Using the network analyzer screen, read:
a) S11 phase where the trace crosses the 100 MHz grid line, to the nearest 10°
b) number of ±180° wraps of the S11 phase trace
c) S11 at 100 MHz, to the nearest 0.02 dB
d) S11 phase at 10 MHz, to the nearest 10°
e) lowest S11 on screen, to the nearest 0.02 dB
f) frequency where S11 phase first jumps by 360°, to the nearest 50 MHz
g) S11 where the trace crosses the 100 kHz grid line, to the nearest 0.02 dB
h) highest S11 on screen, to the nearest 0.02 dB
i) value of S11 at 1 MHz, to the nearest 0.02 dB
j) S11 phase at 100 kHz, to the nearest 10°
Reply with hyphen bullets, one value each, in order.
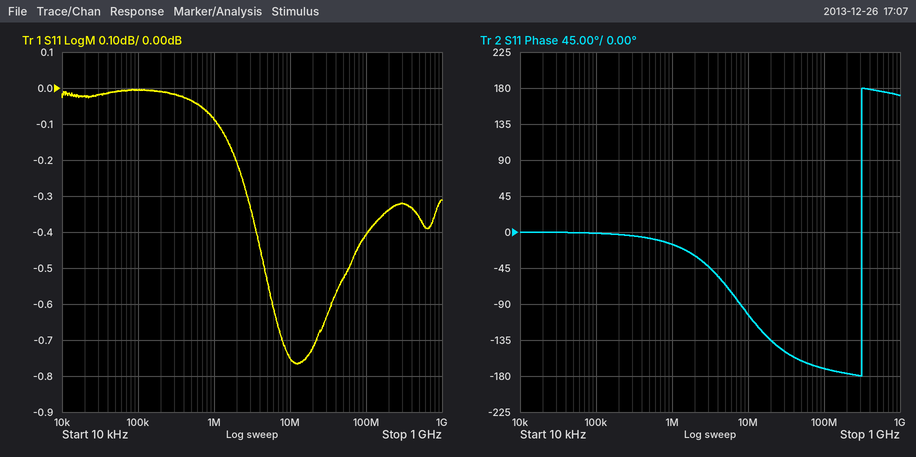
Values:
- -170°
- 1
- -0.40 dB
- -100°
- -0.76 dB
- 300 MHz
- 0.00 dB
- 0.00 dB
- -0.08 dB
- 0°
